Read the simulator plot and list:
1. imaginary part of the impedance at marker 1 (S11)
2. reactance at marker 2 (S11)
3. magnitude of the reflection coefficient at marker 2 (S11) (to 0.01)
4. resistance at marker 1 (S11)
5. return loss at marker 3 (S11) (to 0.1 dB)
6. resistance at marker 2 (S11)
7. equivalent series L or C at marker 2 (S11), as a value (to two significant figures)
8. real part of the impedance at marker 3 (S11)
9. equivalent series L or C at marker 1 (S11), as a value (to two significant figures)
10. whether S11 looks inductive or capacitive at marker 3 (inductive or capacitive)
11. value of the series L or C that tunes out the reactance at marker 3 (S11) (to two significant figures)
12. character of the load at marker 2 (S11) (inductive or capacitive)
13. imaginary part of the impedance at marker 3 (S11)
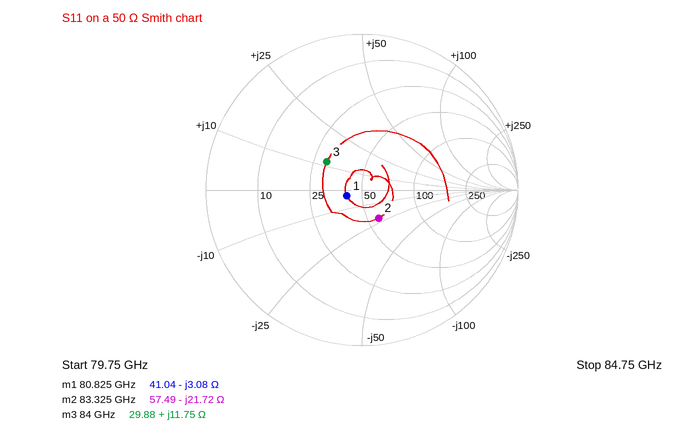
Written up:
-3.08 Ω
-21.72 Ω
0.21
41.04 Ω
10.8 dB
57.49 Ω
88 fF
29.88 Ω
640 fF
inductive
160 fF
capacitive
+11.75 Ω
